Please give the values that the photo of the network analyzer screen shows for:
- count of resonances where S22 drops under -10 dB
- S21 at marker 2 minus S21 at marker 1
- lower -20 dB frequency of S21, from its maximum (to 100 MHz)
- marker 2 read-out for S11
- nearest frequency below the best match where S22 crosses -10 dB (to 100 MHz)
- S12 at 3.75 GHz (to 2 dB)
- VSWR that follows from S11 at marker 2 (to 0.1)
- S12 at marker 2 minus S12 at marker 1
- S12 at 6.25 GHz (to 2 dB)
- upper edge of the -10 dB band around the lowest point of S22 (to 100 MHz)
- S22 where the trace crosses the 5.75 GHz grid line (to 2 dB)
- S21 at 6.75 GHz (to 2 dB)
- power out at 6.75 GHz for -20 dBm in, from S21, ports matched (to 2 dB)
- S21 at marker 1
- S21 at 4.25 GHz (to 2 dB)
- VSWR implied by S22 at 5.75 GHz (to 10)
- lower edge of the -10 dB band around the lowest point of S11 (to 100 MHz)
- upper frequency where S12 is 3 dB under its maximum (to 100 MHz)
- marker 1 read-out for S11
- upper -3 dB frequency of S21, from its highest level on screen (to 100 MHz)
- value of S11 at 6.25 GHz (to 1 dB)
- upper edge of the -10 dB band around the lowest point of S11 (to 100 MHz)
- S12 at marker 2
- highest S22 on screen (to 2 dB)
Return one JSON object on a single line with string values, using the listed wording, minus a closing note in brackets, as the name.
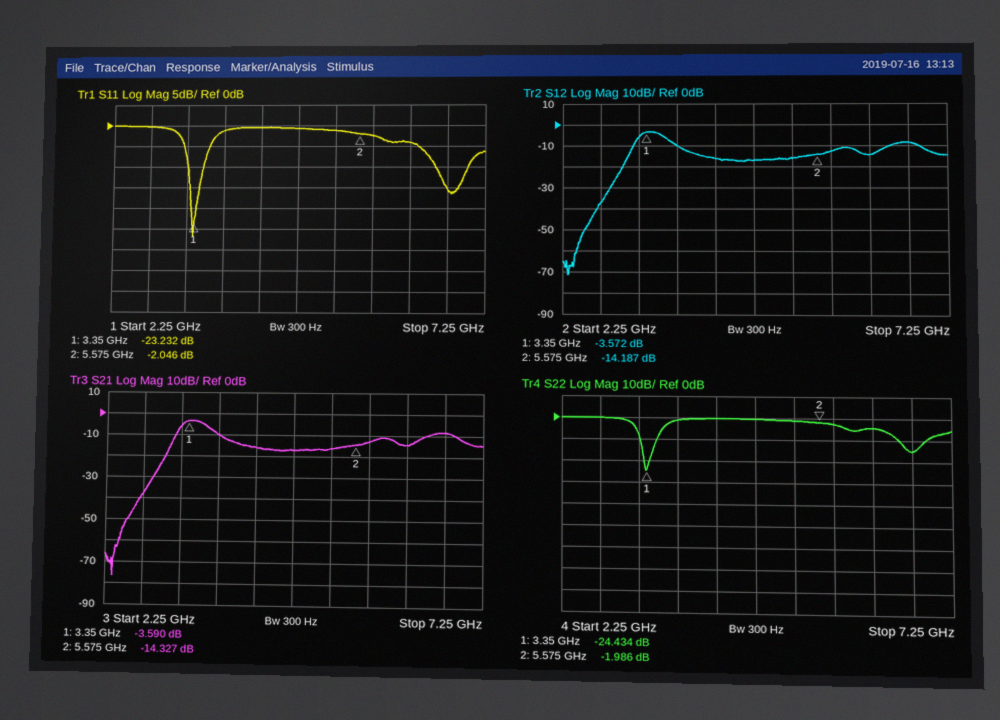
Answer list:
{"count of resonances where S22 drops under -10 dB": "2", "S21 at marker 2 minus S21 at marker 1": "-10.737 dB", "lower -20 dB frequency of S21, from its maximum": "3.0 GHz", "marker 2 read-out for S11": "-2.046 dB", "nearest frequency below the best match where S22 crosses -10 dB": "3.3 GHz", "S12 at 3.75 GHz": "-10 dB", "VSWR that follows from S11 at marker 2": "8.5", "S12 at marker 2 minus S12 at marker 1": "-10.615 dB", "S12 at 6.25 GHz": "-14 dB", "upper edge of the -10 dB band around the lowest point of S22": "3.5 GHz", "S22 where the trace crosses the 5.75 GHz grid line": "-2 dB", "S21 at 6.75 GHz": "-8 dB", "power out at 6.75 GHz for -20 dBm in, from S21, ports matched": "-28 dBm", "S21 at marker 1": "-3.590 dB", "S21 at 4.25 GHz": "-16 dB", "VSWR implied by S22 at 5.75 GHz": "10", "lower edge of the -10 dB band around the lowest point of S11": "3.3 GHz", "upper frequency where S12 is 3 dB under its maximum": "3.6 GHz", "marker 1 read-out for S11": "-23.232 dB", "upper -3 dB frequency of S21, from its highest level on screen": "3.6 GHz", "value of S11 at 6.25 GHz": "-4 dB", "upper edge of the -10 dB band around the lowest point of S11": "3.5 GHz", "S12 at marker 2": "-14.187 dB", "highest S22 on screen": "0 dB"}
